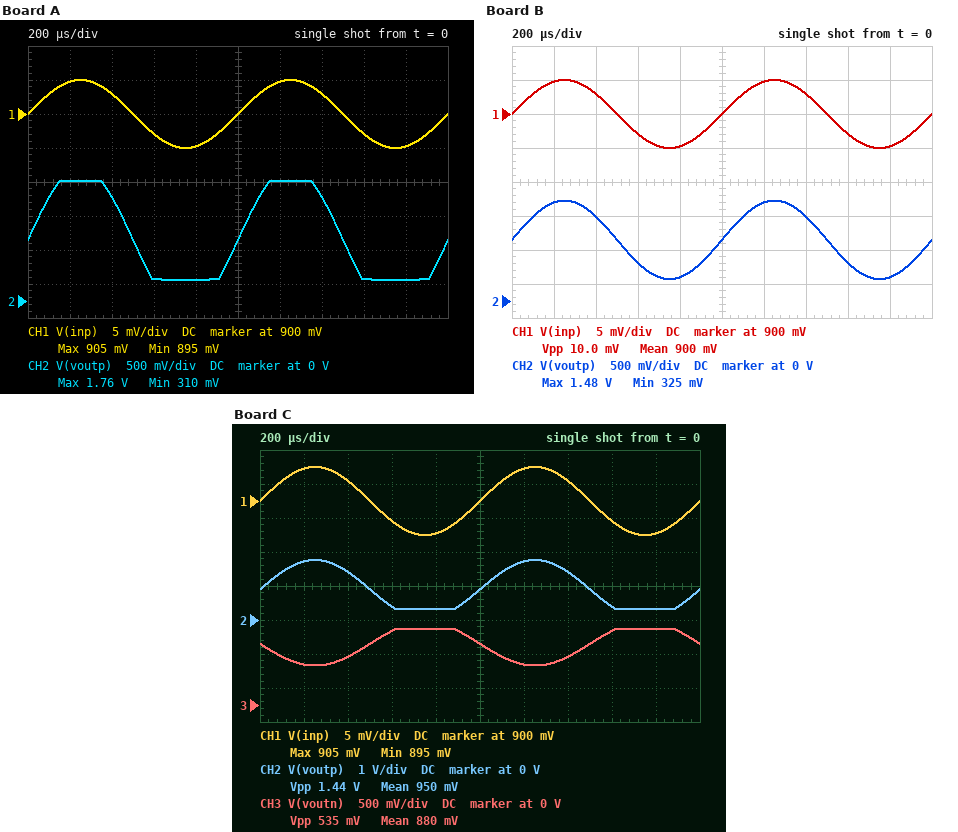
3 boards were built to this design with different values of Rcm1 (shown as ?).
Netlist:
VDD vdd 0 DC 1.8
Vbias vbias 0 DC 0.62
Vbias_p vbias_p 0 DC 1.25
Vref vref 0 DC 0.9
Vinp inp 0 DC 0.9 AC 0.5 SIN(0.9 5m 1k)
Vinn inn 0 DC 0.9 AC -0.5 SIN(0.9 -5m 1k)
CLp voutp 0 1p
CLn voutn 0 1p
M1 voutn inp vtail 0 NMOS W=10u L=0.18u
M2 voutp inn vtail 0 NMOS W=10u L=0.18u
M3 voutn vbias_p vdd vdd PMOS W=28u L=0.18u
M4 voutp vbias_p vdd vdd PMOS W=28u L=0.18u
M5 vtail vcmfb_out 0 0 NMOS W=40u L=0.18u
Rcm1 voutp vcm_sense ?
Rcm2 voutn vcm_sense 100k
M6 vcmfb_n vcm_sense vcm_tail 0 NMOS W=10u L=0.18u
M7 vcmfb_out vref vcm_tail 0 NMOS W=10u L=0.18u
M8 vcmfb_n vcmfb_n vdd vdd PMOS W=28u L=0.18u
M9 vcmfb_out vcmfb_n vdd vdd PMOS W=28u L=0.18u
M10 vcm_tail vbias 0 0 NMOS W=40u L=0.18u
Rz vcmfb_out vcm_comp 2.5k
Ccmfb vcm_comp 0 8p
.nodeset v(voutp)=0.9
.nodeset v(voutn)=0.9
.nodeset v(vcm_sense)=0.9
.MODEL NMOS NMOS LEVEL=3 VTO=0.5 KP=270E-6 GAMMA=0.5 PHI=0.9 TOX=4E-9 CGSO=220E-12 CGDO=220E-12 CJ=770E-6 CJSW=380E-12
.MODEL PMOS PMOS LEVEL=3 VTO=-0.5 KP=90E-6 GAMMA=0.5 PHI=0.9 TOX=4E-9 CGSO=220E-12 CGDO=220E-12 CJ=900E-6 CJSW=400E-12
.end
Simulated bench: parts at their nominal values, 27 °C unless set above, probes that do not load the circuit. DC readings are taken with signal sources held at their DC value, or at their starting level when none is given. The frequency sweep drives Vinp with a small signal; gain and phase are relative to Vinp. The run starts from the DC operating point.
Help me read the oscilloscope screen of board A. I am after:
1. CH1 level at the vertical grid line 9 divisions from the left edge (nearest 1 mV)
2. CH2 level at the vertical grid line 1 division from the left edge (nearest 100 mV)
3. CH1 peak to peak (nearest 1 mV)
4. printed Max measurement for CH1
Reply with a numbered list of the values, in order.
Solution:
1. 895 mV
2. 1.8 V
3. 10 mV
4. 905 mV
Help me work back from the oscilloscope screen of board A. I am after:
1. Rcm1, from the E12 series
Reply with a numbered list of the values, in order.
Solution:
1. 330 kΩ
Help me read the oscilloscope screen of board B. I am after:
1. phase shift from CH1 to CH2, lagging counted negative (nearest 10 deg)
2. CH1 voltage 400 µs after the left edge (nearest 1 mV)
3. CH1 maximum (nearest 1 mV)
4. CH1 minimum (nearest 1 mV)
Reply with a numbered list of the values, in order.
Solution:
1. 0 deg
2. 903 mV
3. 905 mV
4. 895 mV
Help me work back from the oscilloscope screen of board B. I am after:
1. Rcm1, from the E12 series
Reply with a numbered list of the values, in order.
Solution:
1. 180 kΩ
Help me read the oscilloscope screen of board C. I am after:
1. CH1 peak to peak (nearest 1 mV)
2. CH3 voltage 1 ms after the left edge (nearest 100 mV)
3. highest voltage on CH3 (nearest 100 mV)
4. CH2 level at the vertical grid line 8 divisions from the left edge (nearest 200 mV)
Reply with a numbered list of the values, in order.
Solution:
1. 10 mV
2. 900 mV
3. 1.1 V
4. 400 mV
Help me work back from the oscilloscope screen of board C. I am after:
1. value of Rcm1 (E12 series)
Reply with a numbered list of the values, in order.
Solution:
1. 270 kΩ
